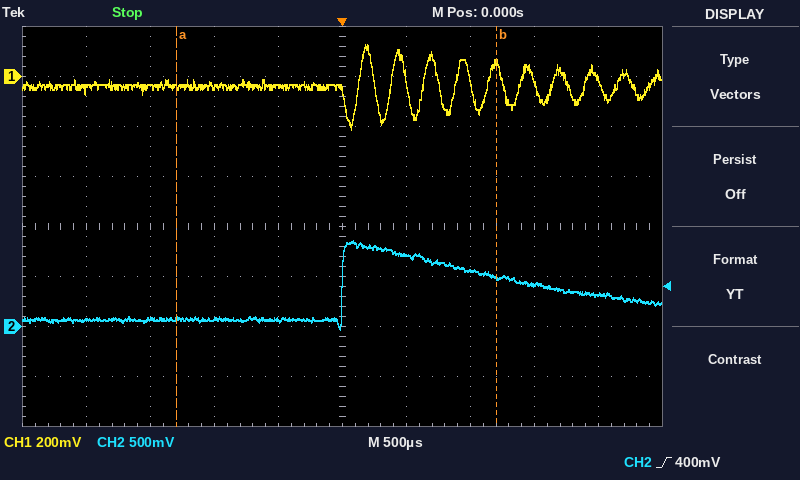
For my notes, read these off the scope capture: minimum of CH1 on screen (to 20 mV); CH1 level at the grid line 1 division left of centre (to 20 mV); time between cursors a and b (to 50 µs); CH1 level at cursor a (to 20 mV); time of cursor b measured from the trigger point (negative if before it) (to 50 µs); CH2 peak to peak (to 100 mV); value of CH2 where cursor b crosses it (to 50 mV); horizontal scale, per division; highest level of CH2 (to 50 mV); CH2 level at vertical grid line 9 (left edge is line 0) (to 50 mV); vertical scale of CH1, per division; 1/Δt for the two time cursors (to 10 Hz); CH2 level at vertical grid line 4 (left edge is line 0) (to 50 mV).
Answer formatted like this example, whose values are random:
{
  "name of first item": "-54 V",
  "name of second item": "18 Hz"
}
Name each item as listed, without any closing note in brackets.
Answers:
{
  "minimum of CH1 on screen": "-220 mV",
  "CH1 level at the grid line 1 division left of centre": "-40 mV",
  "time between cursors a and b": "2.50 ms",
  "CH1 level at cursor a": "-40 mV",
  "time of cursor b measured from the trigger point (negative if before it)": "+1.20 ms",
  "CH2 peak to peak": "900 mV",
  "value of CH2 where cursor b crosses it": "500 mV",
  "horizontal scale, per division": "500 µs",
  "highest level of CH2": "850 mV",
  "CH2 level at vertical grid line 9 (left edge is line 0)": "300 mV",
  "vertical scale of CH1, per division": "200 mV",
  "1/Δt for the two time cursors": "400 Hz",
  "CH2 level at vertical grid line 4 (left edge is line 0)": "50 mV"
}
